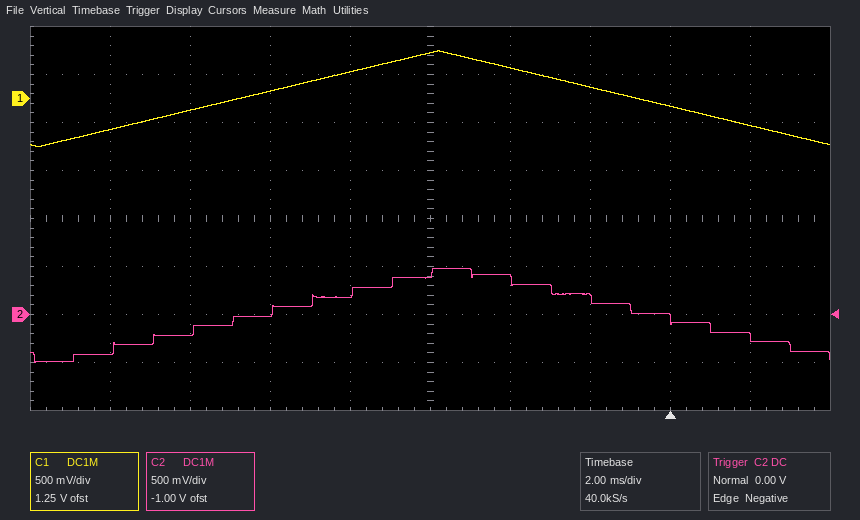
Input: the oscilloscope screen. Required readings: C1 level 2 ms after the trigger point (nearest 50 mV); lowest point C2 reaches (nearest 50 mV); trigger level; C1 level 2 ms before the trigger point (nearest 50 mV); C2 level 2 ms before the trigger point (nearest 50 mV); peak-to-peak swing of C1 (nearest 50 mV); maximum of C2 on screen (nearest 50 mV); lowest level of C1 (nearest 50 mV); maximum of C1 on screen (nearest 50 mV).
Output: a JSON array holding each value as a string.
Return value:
["-300 mV", "-500 mV", "0.00 V", "100 mV", "150 mV", "1.00 V", "500 mV", "-500 mV", "500 mV"]
